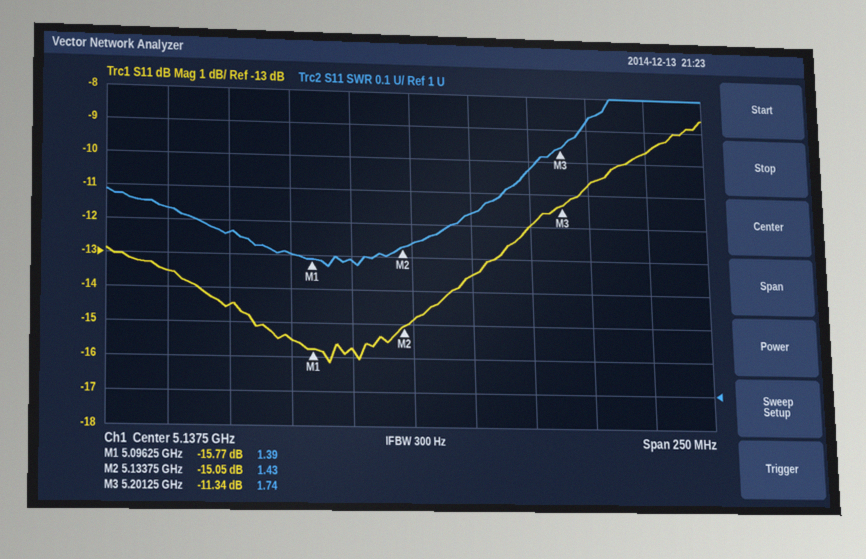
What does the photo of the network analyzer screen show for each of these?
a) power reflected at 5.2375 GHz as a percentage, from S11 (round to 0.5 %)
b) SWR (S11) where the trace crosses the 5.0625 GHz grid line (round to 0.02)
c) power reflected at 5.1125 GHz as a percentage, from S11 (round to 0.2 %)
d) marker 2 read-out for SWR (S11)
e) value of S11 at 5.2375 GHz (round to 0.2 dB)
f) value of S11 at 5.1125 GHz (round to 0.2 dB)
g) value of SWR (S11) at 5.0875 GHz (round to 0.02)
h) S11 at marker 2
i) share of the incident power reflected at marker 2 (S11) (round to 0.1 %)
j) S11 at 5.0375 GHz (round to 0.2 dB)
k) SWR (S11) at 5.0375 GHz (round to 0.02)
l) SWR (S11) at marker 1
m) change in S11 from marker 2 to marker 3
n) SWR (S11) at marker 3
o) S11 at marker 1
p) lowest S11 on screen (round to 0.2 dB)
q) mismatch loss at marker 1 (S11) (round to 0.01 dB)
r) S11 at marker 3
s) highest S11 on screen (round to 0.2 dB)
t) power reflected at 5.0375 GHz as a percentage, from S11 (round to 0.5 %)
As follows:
11.0 %
1.46
2.6 %
1.43
-9.6 dB
-15.8 dB
1.40
-15.05 dB
3.1 %
-13.6 dB
1.54
1.39
3.71 dB
1.74
-15.77 dB
-16.2 dB
0.12 dB
-11.34 dB
-8.6 dB
4.5 %
